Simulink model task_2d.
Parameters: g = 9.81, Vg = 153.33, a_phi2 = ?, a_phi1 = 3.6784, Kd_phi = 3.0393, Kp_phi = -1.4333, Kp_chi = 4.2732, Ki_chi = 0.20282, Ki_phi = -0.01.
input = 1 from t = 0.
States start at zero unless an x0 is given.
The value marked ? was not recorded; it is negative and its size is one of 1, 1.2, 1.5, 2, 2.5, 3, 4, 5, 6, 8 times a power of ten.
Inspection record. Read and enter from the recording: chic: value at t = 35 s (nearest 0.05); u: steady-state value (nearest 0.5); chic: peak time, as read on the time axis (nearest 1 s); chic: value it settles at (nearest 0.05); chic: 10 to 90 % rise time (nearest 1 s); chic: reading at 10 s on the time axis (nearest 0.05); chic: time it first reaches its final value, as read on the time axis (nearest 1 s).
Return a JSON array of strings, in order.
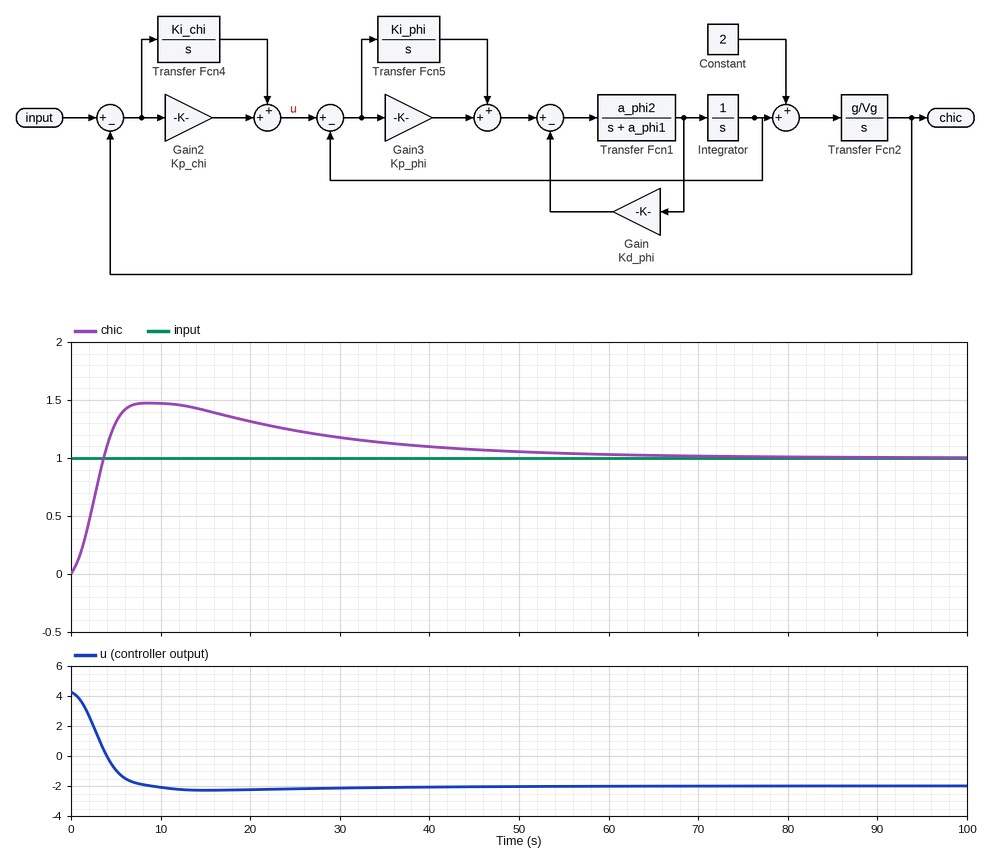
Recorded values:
["1.15", "-2.0", "9 s", "1.00", "3 s", "1.45", "4 s"]
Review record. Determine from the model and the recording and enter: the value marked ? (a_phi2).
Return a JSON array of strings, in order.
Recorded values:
["-0.8"]
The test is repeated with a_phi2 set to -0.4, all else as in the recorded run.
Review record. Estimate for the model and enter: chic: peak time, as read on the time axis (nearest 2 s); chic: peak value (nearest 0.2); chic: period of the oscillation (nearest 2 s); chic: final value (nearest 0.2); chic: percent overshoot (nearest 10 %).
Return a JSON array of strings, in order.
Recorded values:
["12 s", "2.0", "26 s", "1.0", "90 %"]
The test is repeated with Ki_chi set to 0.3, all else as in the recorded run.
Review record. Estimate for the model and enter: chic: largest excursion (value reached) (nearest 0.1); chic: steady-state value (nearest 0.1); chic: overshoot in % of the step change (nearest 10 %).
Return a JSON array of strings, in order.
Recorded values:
["1.5", "1.0", "50 %"]
